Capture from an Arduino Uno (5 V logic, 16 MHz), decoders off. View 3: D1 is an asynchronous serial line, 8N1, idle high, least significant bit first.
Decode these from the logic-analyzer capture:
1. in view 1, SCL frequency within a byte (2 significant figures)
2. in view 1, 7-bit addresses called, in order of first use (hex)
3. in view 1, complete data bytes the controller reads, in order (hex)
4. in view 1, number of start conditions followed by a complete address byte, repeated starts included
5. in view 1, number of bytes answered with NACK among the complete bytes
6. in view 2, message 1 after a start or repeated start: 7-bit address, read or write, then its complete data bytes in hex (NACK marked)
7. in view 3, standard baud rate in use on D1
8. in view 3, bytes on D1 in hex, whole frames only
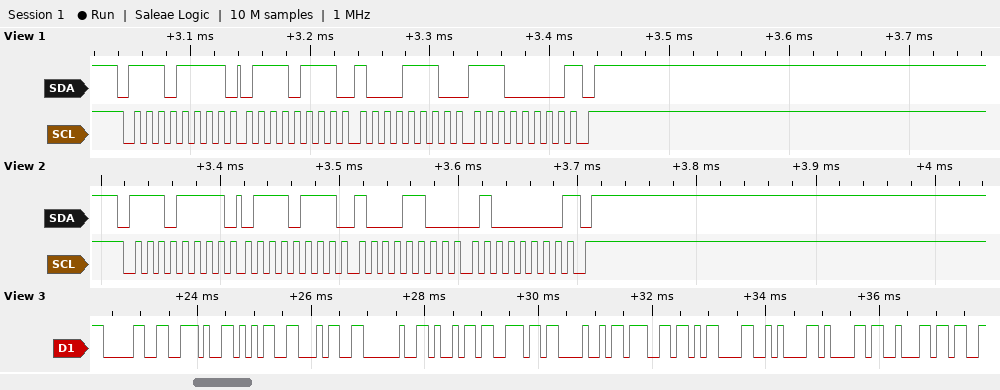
100 kHz
0x77
77 8E E0
1
1
0x77 read: 77 8C 40 NACK
9600 baud
30 2E 35 34 20 69 6E 48 67 0D 0A 61 62
